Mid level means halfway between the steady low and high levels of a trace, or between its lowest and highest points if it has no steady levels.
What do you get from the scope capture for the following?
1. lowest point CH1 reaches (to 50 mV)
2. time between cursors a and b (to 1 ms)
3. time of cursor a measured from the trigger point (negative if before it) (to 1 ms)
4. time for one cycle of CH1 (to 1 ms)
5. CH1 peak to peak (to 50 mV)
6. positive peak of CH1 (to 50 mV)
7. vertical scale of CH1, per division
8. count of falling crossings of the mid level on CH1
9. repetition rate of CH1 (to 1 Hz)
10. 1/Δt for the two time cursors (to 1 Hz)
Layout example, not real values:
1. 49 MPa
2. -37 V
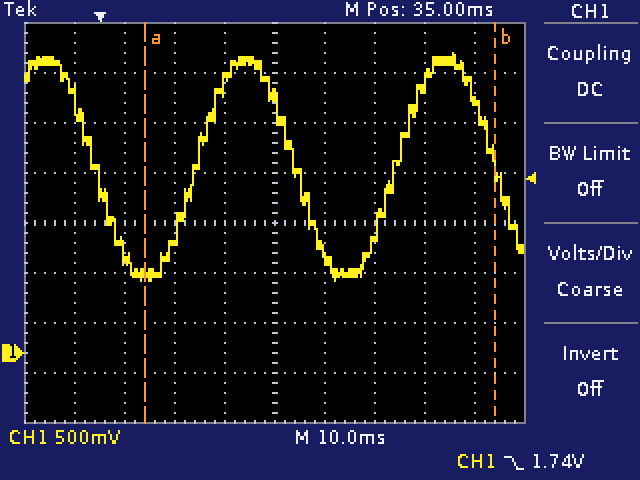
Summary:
1. 700 mV
2. 70 ms
3. +9 ms
4. 40 ms
5. 2.30 V
6. 3.00 V
7. 500 mV
8. 3
9. 25 Hz
10. 14 Hz
